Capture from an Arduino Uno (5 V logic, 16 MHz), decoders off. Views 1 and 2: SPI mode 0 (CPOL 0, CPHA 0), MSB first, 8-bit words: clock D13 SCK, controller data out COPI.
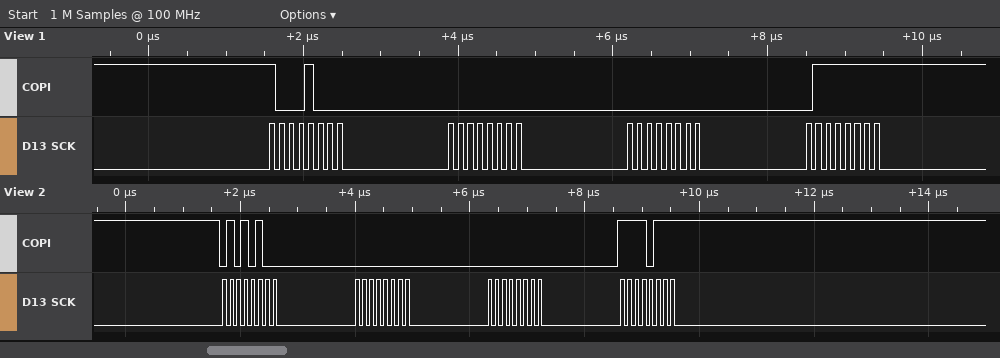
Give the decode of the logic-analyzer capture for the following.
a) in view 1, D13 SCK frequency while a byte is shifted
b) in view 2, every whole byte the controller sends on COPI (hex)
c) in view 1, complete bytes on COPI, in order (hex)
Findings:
8 MHz
54 00 00 F7
88 00 00 7F
